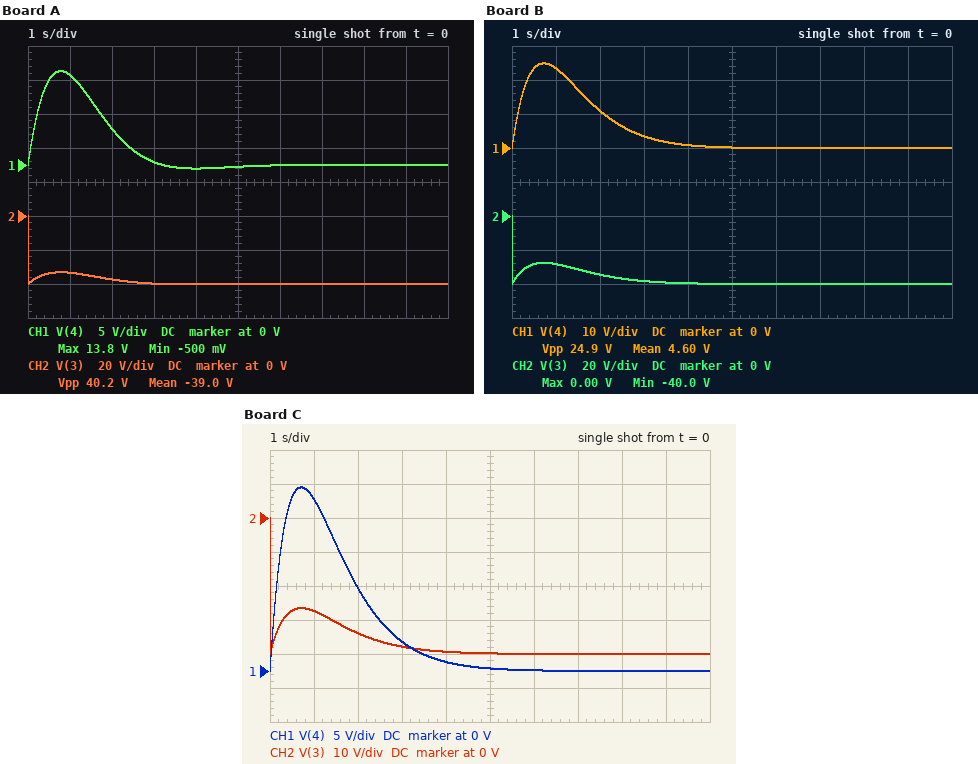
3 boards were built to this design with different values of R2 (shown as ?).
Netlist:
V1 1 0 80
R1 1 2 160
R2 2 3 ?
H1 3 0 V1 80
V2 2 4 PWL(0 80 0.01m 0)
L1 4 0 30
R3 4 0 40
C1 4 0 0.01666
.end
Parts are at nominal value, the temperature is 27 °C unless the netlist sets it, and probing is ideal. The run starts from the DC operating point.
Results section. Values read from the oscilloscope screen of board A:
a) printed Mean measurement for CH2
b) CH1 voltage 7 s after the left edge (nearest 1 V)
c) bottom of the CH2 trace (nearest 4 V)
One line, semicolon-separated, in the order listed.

-39.0 V; 0 V; -40 V
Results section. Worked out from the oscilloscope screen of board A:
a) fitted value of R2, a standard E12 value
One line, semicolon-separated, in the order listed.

180 Ω
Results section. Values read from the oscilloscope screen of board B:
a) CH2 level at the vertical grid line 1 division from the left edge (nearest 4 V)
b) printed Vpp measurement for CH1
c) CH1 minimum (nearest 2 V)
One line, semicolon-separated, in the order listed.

-28 V; 24.9 V; 0 V
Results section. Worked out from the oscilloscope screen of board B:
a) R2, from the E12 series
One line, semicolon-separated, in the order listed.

39 Ω
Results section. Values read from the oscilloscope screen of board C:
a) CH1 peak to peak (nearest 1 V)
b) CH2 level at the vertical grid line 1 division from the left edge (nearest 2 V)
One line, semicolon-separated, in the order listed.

27 V; -28 V
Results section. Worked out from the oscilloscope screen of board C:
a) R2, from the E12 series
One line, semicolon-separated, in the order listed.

33 Ω
